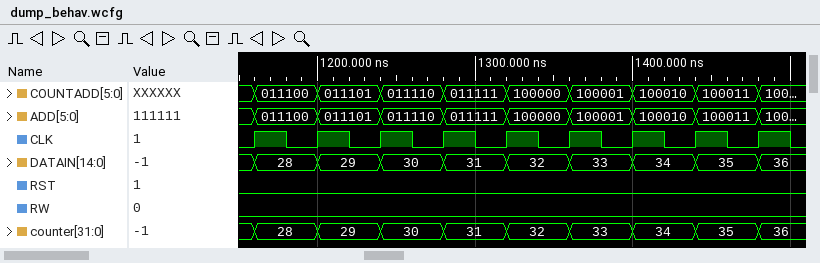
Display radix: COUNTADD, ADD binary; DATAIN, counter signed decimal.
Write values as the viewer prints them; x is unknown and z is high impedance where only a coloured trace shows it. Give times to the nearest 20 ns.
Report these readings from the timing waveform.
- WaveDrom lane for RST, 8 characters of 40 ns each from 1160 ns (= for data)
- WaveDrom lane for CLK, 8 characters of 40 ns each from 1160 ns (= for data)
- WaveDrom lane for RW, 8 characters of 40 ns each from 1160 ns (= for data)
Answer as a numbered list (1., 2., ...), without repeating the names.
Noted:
1. {name: 'RST', wave: '0.......'}
2. {name: 'CLK', wave: 'p.......'}
3. {name: 'RW', wave: '0.......'}
